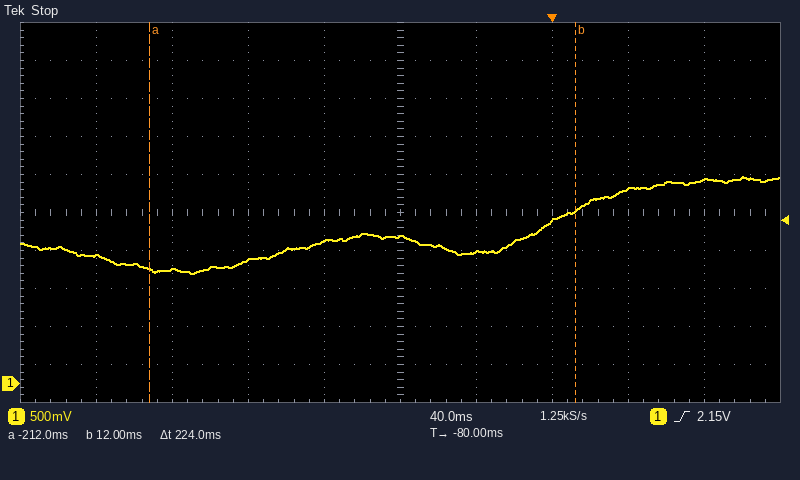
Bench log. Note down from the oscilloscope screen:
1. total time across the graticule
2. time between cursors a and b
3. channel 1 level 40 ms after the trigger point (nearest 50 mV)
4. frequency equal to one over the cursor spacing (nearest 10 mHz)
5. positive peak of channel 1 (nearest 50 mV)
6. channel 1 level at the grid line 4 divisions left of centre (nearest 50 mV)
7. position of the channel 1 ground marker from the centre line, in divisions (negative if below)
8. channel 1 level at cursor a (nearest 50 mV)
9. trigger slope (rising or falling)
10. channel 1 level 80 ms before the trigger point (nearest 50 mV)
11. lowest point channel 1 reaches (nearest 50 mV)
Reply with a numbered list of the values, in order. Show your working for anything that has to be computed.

1. 400 ms
2. 224 ms
3. 2.55 V
4. 1 / 224 ms ≈ 4.46 Hz
5. 2.70 V
6. 1.70 V
7. -4.5 div
8. 1.50 V
9. rising
10. 1.95 V
11. 1.45 V
